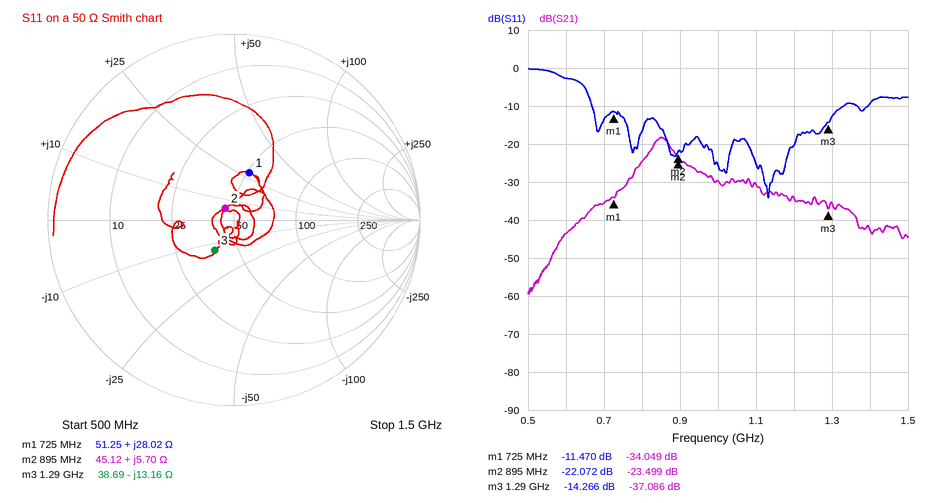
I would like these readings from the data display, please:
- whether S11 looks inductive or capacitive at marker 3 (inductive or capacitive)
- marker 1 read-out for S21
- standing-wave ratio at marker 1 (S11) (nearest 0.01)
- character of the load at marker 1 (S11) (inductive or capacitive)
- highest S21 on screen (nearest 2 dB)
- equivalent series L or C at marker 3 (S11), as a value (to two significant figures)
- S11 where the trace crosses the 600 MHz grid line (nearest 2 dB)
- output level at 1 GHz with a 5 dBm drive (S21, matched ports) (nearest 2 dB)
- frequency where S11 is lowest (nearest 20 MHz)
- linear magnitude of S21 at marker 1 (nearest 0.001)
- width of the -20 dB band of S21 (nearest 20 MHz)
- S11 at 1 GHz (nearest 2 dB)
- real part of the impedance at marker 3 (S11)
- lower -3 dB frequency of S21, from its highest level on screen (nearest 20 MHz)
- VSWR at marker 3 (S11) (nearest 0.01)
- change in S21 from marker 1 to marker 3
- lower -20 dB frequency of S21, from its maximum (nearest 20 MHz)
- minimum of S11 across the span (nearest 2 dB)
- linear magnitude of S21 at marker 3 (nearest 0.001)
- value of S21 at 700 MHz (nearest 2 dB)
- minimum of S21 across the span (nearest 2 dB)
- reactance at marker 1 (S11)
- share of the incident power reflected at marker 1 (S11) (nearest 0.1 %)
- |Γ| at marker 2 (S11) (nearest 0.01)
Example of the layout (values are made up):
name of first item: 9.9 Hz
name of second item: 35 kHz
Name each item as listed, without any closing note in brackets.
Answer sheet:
whether S11 looks inductive or capacitive at marker 3: capacitive
marker 1 read-out for S21: -34.049 dB
standing-wave ratio at marker 1 (S11): 1.73
character of the load at marker 1 (S11): inductive
highest S21 on screen: -18 dB
equivalent series L or C at marker 3 (S11), as a value: 9.4 pF
S11 where the trace crosses the 600 MHz grid line: -2 dB
output level at 1 GHz with a 5 dBm drive (S21, matched ports): -24 dBm
frequency where S11 is lowest: 1.14 GHz
linear magnitude of S21 at marker 1: 0.020
width of the -20 dB band of S21: 700 MHz
S11 at 1 GHz: -26 dB
real part of the impedance at marker 3: 38.69 Ω
lower -3 dB frequency of S21, from its highest level on screen: 820 MHz
VSWR at marker 3 (S11): 1.48
change in S21 from marker 1 to marker 3: -3.037 dB
lower -20 dB frequency of S21, from its maximum: 660 MHz
minimum of S11 across the span: -34 dB
linear magnitude of S21 at marker 3: 0.014
value of S21 at 700 MHz: -36 dB
minimum of S21 across the span: -60 dB
reactance at marker 1: +28.02 Ω
share of the incident power reflected at marker 1 (S11): 7.1 %
|Γ| at marker 2 (S11): 0.08
